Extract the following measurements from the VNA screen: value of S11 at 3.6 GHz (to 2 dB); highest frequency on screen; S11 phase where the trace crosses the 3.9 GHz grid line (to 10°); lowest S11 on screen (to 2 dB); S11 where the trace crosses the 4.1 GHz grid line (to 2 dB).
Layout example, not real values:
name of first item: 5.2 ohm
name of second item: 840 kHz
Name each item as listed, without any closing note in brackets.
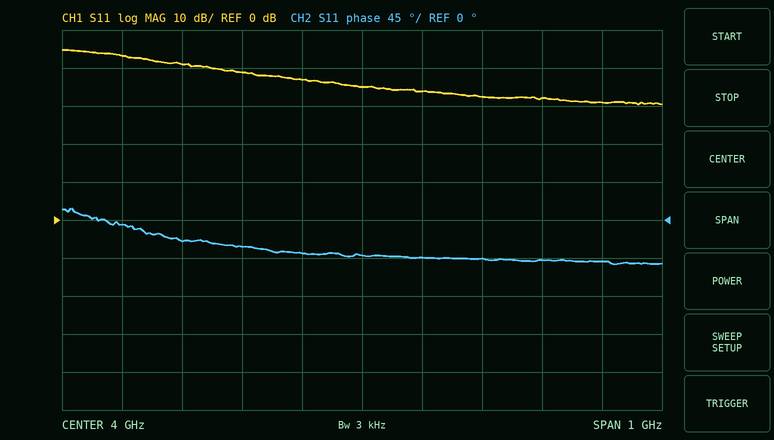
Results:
value of S11 at 3.6 GHz: 44 dB
highest frequency on screen: 4.5 GHz
S11 phase where the trace crosses the 3.9 GHz grid line: -40°
lowest S11 on screen: 30 dB
S11 where the trace crosses the 4.1 GHz grid line: 34 dB
